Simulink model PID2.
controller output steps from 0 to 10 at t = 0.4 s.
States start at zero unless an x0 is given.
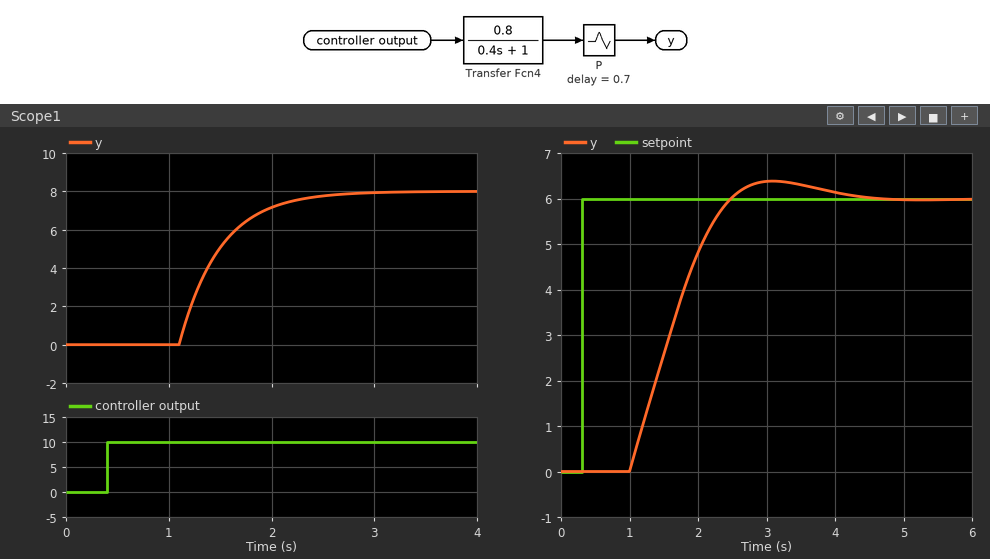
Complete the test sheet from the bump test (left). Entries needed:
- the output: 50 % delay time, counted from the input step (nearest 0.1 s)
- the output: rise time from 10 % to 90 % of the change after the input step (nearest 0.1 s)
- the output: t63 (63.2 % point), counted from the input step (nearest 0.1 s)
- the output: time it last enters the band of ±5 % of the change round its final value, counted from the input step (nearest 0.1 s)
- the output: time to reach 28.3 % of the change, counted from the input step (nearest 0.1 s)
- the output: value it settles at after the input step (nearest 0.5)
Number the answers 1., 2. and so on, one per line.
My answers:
1. 1.0 s
2. 0.9 s
3. 1.1 s
4. 1.9 s
5. 0.8 s
6. 8.0
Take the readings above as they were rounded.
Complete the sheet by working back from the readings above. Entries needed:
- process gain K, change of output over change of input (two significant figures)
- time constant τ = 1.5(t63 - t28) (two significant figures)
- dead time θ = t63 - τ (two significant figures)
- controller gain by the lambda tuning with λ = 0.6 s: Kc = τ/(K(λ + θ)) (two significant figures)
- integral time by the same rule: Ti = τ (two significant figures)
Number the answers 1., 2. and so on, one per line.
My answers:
1. 0.80
2. 0.45 s
3. 0.65 s
4. 0.45
5. 0.45 s
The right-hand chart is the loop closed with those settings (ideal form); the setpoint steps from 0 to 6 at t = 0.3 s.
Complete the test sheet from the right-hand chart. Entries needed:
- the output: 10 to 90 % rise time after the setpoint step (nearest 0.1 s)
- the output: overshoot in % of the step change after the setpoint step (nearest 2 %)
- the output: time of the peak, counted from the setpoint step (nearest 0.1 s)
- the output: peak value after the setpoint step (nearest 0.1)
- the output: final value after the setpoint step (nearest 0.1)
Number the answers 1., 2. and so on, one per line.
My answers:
1. 1.1 s
2. 6 %
3. 2.8 s
4. 6.4
5. 6.0
